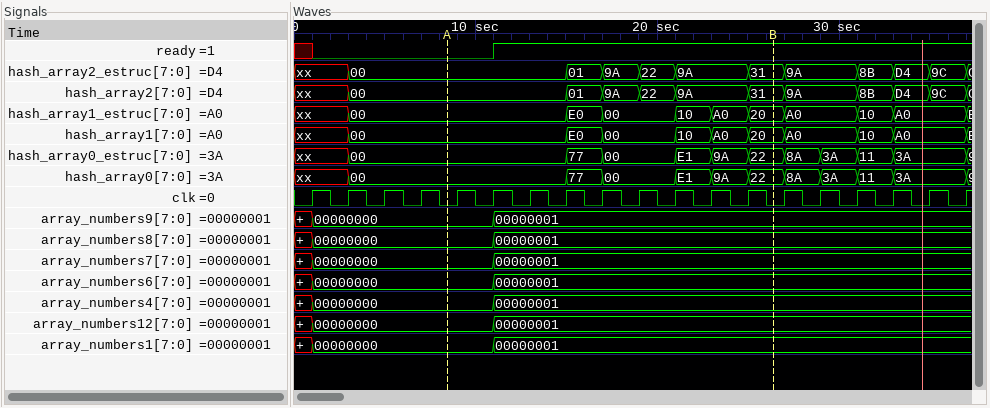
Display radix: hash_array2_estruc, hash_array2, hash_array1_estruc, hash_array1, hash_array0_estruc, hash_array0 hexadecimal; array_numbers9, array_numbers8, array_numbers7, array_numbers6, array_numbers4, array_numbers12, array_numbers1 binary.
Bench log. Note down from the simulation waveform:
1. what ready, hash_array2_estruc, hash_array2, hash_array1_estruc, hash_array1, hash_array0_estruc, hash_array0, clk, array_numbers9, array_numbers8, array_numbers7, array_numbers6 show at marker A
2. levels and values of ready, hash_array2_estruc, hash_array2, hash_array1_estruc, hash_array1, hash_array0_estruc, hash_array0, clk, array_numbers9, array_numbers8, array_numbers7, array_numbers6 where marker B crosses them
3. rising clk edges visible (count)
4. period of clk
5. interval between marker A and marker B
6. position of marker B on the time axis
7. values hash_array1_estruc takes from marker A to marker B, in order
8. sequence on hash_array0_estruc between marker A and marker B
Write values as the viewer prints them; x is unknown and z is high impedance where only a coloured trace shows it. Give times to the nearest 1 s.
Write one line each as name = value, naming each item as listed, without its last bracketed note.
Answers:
what ready, hash_array2_estruc, hash_array2, hash_array1_estruc, hash_array1, hash_array0_estruc, hash_array0, clk, array_numbers9, array_numbers8, array_numbers7, array_numbers6 show at marker A = ready=0, hash_array2_estruc=00, hash_array2=00, hash_array1_estruc=00, hash_array1=00, hash_array0_estruc=00, hash_array0=00, clk=0, array_numbers9=00000000, array_numbers8=00000000, array_numbers7=00000000, array_numbers6=00000000
levels and values of ready, hash_array2_estruc, hash_array2, hash_array1_estruc, hash_array1, hash_array0_estruc, hash_array0, clk, array_numbers9, array_numbers8, array_numbers7, array_numbers6 where marker B crosses them = ready=1, hash_array2_estruc=31, hash_array2=31, hash_array1_estruc=20, hash_array1=20, hash_array0_estruc=22, hash_array0=22, clk=0, array_numbers9=00000001, array_numbers8=00000001, array_numbers7=00000001, array_numbers6=00000001
rising clk edges visible = 19
period of clk = 2 s
interval between marker A and marker B = 18 s
position of marker B on the time axis = 26 s
values hash_array1_estruc takes from marker A to marker B, in order = 00, E0, 00, 10, A0, 20
sequence on hash_array0_estruc between marker A and marker B = 00, 77, 00, E1, 9A, 22
